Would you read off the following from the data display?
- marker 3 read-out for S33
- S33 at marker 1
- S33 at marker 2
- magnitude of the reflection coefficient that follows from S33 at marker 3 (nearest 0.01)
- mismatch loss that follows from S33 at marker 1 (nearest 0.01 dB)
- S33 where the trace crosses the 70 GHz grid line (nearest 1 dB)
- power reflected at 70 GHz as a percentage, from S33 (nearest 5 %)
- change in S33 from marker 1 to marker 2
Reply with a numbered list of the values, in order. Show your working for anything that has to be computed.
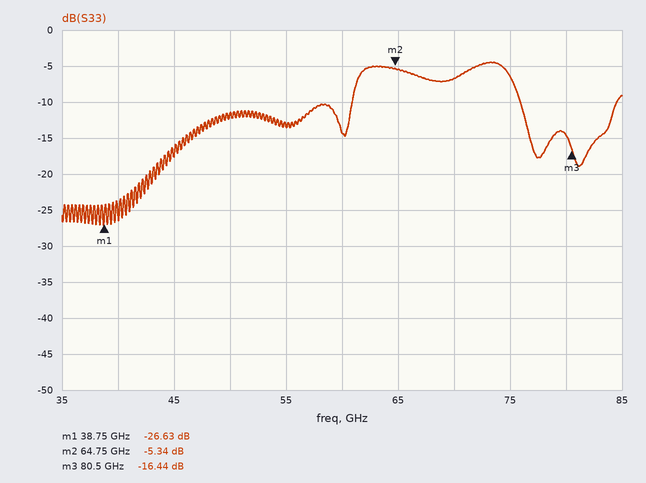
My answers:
1. -16.44 dB
2. -26.63 dB
3. -5.34 dB
4. 10^(-16.44/20) ≈ 0.15
5. −10 log10(1 − 10^(-26.63/10)) ≈ 0.01 dB
6. -7 dB
7. 10^(-7/10) ≈ 20 %
8. -5.34 − (-26.63) = 21.29 dB
